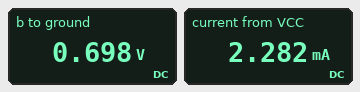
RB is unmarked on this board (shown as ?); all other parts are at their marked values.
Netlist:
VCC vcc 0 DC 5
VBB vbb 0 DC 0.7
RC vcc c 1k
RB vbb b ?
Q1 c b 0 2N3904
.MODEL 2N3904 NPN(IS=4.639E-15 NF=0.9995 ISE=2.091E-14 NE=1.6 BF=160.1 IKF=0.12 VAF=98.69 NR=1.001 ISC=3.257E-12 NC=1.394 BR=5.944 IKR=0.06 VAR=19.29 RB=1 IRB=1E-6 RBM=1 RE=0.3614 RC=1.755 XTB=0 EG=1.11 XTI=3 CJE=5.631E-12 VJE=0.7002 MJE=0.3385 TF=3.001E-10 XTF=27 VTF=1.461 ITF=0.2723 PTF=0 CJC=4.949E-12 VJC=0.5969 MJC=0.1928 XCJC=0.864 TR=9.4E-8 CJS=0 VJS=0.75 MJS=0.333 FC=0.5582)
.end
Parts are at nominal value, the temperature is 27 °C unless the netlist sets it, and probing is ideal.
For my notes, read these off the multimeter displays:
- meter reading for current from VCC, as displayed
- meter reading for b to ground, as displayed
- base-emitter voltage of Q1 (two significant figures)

2.282 mA
0.698 V
700 mV
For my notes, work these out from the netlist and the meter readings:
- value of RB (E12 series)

150 Ω
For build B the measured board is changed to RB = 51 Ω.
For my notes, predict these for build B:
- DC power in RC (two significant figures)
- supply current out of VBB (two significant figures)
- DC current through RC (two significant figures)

5.8 mW
16 µA
2.4 mA
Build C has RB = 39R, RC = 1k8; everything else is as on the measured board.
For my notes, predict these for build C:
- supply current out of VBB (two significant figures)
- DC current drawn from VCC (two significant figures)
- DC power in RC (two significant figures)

16 µA
2.4 mA
10 mW
